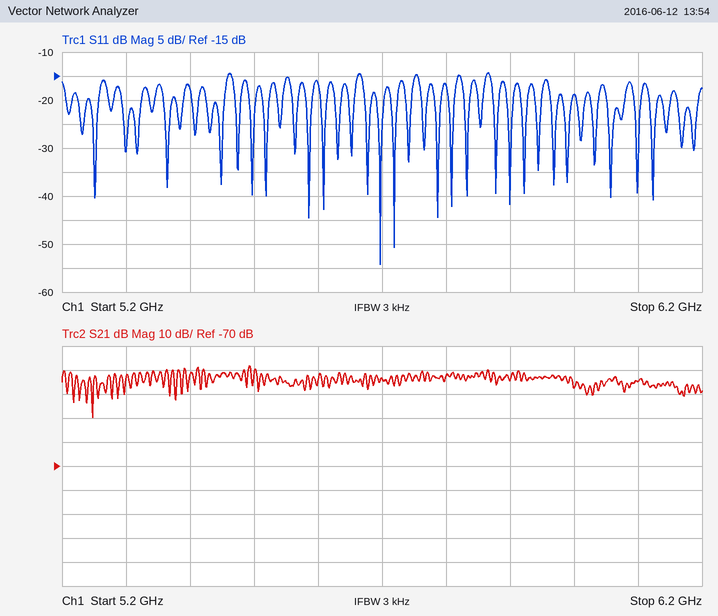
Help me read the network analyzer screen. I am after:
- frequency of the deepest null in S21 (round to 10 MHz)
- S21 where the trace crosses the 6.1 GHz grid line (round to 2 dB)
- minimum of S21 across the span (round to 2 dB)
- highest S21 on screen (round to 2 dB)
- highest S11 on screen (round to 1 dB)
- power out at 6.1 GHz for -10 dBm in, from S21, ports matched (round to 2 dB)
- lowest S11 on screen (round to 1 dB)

5.25 GHz
-34 dB
-50 dB
-28 dB
-14 dB
-44 dBm
-54 dB
